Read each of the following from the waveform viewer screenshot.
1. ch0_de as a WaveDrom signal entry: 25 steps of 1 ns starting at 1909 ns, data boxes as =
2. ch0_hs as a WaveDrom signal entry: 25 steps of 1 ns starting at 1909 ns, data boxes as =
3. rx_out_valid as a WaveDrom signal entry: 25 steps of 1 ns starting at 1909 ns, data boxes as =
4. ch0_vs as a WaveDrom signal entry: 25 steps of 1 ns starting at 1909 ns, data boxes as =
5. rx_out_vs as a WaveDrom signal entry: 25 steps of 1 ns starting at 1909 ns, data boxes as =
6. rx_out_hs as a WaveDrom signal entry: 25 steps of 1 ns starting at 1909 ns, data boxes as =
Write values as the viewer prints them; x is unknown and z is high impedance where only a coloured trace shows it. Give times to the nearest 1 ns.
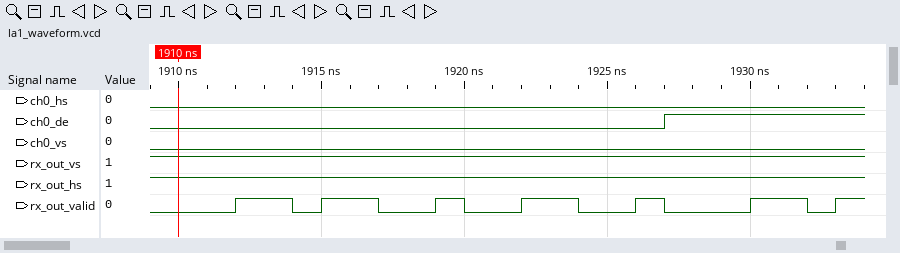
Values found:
{name: 'ch0_de', wave: '0.................1......'}
{name: 'ch0_hs', wave: '0........................'}
{name: 'rx_out_valid', wave: '0..1.01.0.10.1.0.10..1.01'}
{name: 'ch0_vs', wave: '0........................'}
{name: 'rx_out_vs', wave: '1........................'}
{name: 'rx_out_hs', wave: '1........................'}
